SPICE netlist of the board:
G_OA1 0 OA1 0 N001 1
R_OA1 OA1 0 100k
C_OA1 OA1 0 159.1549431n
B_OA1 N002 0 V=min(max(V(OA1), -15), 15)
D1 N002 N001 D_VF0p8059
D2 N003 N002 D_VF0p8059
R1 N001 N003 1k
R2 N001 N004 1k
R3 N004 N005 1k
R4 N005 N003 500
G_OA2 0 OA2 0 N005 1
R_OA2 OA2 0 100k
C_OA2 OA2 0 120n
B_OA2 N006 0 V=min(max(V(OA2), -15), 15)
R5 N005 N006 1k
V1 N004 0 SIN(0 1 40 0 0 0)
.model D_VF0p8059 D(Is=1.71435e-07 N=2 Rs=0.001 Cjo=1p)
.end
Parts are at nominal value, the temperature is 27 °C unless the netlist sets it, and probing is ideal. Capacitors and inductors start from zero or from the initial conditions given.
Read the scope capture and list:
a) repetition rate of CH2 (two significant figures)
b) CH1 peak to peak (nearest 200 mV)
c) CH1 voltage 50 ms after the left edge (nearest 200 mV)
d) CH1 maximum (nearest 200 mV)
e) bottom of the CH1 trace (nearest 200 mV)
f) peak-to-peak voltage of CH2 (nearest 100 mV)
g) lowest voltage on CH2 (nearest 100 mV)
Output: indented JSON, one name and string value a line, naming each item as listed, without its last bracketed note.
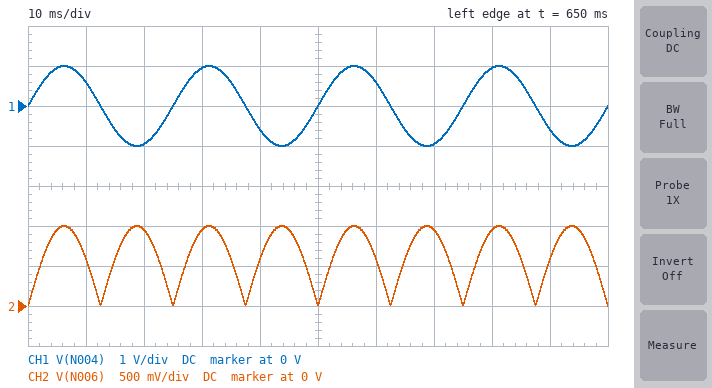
{
  "repetition rate of CH2": "80 Hz",
  "CH1 peak to peak": "2.0 V",
  "CH1 voltage 50 ms after the left edge": "0 V",
  "CH1 maximum": "1.0 V",
  "bottom of the CH1 trace": "-1.0 V",
  "peak-to-peak voltage of CH2": "1.0 V",
  "lowest voltage on CH2": "0 V"
}
